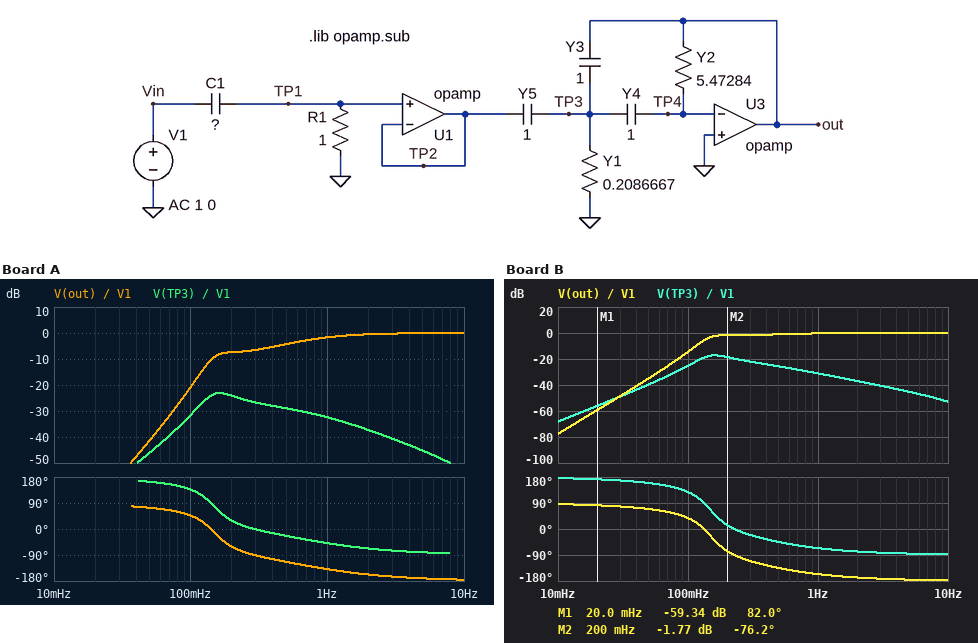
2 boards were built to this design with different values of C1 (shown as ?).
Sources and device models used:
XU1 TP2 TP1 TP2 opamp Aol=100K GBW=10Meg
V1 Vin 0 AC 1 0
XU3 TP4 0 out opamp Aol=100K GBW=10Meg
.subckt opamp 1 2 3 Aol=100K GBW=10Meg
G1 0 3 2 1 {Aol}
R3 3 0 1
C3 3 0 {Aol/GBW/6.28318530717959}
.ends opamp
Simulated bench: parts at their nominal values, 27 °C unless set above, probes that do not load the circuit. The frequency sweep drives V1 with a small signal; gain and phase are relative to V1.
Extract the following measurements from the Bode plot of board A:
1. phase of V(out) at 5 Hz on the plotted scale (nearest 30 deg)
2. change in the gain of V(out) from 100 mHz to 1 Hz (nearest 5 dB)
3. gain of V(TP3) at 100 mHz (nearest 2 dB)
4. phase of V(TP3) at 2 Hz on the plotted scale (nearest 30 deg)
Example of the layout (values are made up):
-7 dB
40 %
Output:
-180 deg
20 dB
-32 dB
-60 deg
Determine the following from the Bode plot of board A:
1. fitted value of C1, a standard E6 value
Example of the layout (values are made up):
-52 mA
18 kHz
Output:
220 mF
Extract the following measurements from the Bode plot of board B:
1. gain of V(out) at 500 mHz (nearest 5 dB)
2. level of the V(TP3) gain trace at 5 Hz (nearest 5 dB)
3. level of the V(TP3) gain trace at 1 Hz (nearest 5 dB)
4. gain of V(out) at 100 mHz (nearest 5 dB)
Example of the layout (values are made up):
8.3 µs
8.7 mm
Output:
0 dB
-45 dB
-30 dB
-15 dB
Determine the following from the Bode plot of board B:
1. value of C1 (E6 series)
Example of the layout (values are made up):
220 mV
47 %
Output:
470 mF
